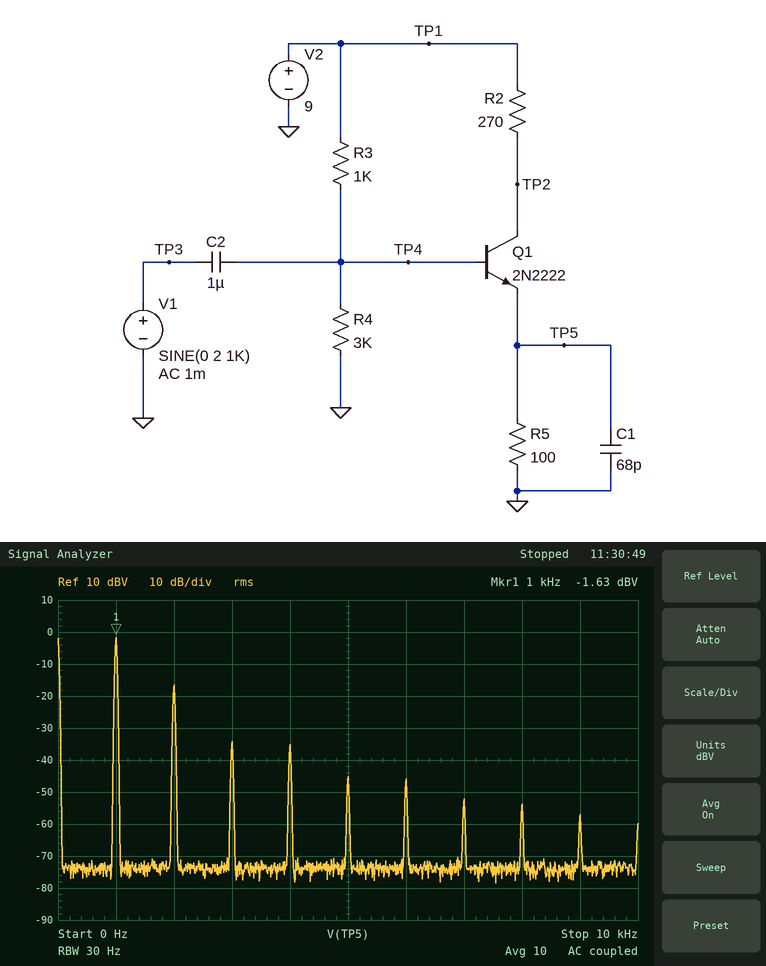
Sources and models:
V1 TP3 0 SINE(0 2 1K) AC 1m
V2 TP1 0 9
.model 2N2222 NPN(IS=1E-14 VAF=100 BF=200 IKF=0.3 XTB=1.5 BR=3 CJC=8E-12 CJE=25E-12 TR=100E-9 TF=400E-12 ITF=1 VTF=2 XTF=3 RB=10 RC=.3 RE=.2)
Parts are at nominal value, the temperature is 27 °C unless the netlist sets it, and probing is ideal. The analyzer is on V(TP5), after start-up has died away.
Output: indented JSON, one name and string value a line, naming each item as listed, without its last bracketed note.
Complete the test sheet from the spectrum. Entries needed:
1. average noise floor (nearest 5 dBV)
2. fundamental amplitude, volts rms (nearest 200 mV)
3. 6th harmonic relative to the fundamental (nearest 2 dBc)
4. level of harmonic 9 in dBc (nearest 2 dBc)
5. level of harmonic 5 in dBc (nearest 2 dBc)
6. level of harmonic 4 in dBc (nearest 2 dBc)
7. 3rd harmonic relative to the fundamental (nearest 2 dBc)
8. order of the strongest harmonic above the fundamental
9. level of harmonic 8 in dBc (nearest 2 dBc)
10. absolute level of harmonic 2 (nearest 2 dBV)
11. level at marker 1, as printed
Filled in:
{
  "average noise floor": "-75 dBV",
  "fundamental amplitude, volts rms": "800 mV",
  "6th harmonic relative to the fundamental": "-44 dBc",
  "level of harmonic 9 in dBc": "-56 dBc",
  "level of harmonic 5 in dBc": "-44 dBc",
  "level of harmonic 4 in dBc": "-34 dBc",
  "3rd harmonic relative to the fundamental": "-32 dBc",
  "order of the strongest harmonic above the fundamental": "2",
  "level of harmonic 8 in dBc": "-52 dBc",
  "absolute level of harmonic 2": "-16 dBV",
  "level at marker 1, as printed": "-1.63 dBV"
}
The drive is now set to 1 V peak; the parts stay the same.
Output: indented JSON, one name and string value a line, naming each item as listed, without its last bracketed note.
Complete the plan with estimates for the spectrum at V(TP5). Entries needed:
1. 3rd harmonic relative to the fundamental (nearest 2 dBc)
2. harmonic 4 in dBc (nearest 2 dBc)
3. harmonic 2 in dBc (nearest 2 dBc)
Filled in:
{
  "3rd harmonic relative to the fundamental": "-30 dBc",
  "harmonic 4 in dBc": "-36 dBc",
  "harmonic 2 in dBc": "-24 dBc"
}
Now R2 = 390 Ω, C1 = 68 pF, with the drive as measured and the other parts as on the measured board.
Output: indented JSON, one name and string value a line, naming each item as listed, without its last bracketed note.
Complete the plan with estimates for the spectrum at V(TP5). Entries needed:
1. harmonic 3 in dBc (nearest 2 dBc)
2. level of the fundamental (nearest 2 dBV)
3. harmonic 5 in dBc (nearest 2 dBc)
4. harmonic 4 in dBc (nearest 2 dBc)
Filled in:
{
  "harmonic 3 in dBc": "-30 dBc",
  "level of the fundamental": "-2 dBV",
  "harmonic 5 in dBc": "-40 dBc",
  "harmonic 4 in dBc": "-36 dBc"
}
